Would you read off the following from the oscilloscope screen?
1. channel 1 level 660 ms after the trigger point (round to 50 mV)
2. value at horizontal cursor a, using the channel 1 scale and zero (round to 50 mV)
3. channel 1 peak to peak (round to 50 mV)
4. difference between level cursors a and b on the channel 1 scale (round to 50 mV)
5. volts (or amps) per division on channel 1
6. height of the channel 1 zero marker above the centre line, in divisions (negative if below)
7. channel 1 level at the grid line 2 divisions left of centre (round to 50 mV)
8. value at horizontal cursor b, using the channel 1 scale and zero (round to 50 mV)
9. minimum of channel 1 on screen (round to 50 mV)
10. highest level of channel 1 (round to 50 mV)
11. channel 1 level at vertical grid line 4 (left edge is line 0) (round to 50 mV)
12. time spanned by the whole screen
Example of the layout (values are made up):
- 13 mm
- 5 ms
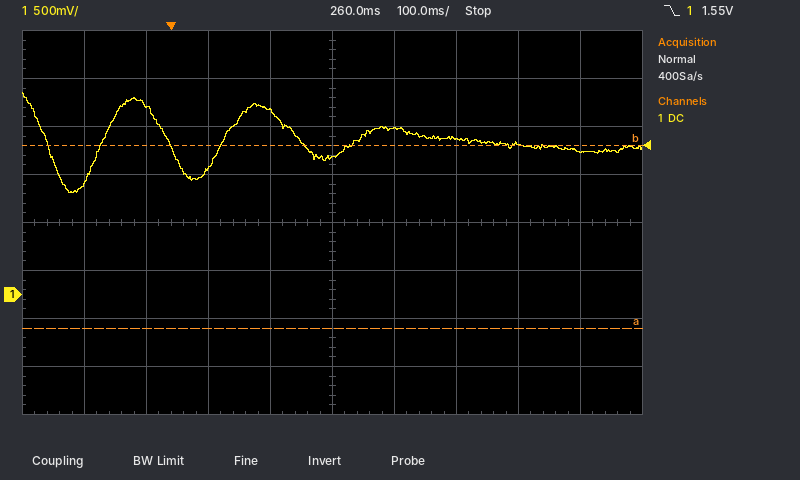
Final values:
- 1.50 V
- -350 mV
- 1.05 V
- 1.90 V
- 500 mV
- -1.5 div
- 1.30 V
- 1.55 V
- 1.05 V
- 2.10 V
- 1.90 V
- 1 s
